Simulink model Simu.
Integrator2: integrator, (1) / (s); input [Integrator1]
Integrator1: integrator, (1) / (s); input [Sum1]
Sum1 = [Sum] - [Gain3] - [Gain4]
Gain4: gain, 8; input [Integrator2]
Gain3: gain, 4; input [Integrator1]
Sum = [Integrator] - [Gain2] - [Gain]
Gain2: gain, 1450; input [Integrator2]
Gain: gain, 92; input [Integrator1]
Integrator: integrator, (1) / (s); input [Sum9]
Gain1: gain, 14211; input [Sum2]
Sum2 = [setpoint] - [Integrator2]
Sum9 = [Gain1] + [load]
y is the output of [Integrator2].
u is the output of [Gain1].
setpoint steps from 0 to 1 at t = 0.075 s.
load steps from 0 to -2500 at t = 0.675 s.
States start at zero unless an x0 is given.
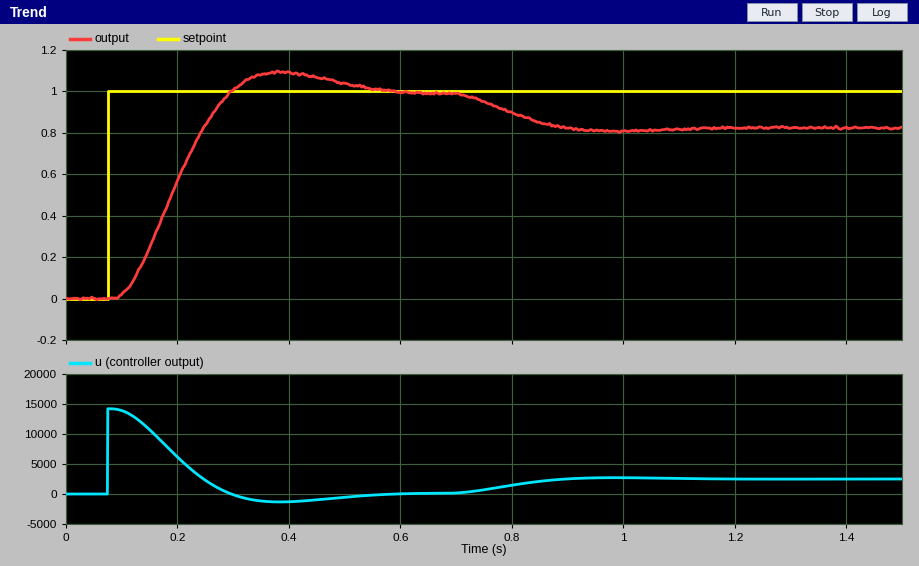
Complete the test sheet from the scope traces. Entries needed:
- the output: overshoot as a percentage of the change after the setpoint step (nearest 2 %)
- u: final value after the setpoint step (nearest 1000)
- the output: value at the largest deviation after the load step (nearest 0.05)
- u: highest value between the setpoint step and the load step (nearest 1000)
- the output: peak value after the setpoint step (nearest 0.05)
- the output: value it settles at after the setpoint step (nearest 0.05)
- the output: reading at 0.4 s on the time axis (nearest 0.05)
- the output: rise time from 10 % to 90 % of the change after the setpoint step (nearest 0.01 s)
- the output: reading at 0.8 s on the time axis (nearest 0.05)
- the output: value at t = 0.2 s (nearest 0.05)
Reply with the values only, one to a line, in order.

10 %
0
0.80
14000
1.10
1.00
1.10
0.14 s
0.90
0.55
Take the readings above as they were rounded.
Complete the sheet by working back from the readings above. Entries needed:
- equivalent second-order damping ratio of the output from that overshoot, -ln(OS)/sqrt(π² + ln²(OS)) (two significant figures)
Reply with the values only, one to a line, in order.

0.59
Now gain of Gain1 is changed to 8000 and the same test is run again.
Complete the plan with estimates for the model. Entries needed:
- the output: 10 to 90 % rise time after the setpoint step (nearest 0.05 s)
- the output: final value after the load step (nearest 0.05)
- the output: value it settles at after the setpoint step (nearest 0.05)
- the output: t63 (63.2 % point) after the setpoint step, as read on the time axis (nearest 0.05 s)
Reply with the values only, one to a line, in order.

0.25 s
0.70
1.00
0.30 s
